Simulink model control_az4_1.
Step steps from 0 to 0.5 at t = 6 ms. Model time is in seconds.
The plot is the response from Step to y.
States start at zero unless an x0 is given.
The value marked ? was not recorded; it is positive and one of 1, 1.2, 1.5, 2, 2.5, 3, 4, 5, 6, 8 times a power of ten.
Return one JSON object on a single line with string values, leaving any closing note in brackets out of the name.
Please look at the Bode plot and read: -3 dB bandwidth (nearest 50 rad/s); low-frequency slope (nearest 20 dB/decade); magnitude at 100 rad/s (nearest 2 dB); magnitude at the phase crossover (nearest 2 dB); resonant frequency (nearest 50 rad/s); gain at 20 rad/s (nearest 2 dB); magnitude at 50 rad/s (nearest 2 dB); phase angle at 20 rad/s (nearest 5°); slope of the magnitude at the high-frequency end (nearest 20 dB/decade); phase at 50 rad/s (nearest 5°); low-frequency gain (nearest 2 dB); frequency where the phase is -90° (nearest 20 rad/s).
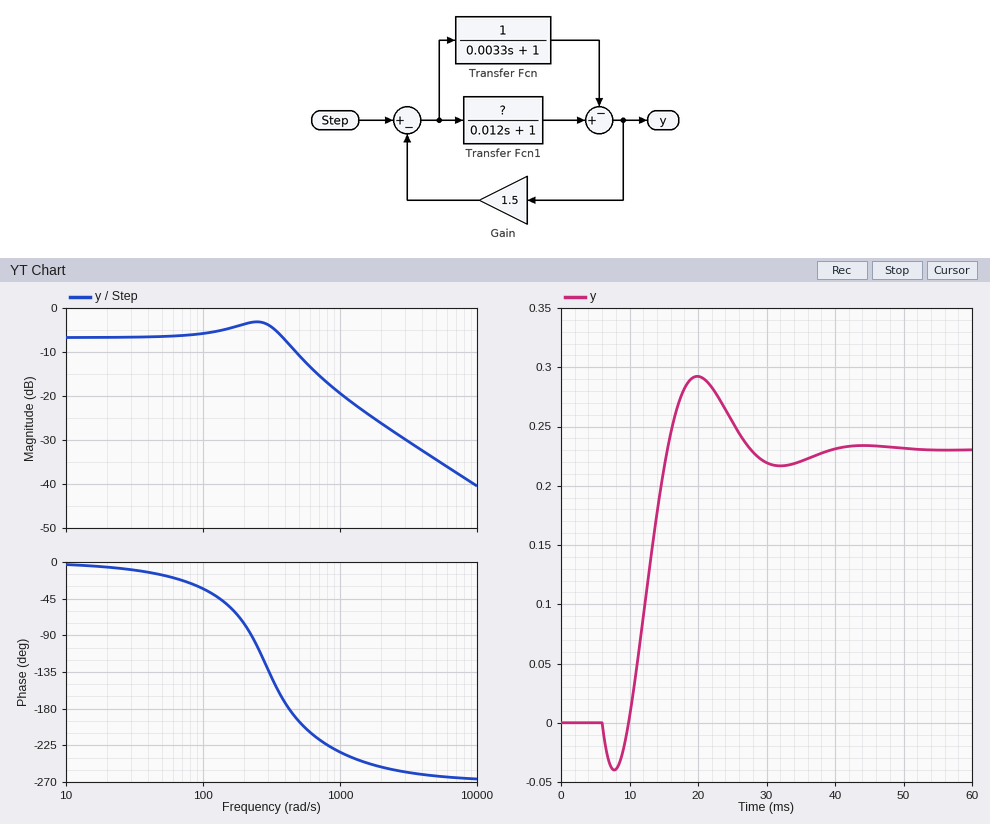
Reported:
{"-3 dB bandwidth": "450 rad/s", "low-frequency slope": "0 dB/decade", "magnitude at 100 rad/s": "-6 dB", "magnitude at the phase crossover": "-8 dB", "resonant frequency": "250 rad/s", "gain at 20 rad/s": "-6 dB", "magnitude at 50 rad/s": "-6 dB", "phase angle at 20 rad/s": "-5°", "slope of the magnitude at the high-frequency end": "-20 dB/decade", "phase at 50 rad/s": "-15°", "low-frequency gain": "-6 dB", "frequency where the phase is -90°": "220 rad/s"}
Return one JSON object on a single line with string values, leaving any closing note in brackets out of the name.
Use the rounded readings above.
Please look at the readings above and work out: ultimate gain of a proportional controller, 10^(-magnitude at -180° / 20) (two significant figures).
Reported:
{"ultimate gain of a proportional controller, 10^(-magnitude at -180° / 20)": "2.5"}
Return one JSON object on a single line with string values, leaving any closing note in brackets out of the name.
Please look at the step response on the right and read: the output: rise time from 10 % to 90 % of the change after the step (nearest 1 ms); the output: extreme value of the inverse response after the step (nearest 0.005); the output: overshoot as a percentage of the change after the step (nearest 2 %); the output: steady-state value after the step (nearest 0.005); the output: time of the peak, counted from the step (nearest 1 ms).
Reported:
{"the output: rise time from 10 % to 90 % of the change after the step": "4 ms", "the output: extreme value of the inverse response after the step": "-0.040", "the output: overshoot as a percentage of the change after the step": "26 %", "the output: steady-state value after the step": "0.230", "the output: time of the peak, counted from the step": "14 ms"}
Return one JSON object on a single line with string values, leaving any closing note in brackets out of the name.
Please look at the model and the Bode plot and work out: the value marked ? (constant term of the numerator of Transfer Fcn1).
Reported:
{"the value marked ?": "2.5"}
